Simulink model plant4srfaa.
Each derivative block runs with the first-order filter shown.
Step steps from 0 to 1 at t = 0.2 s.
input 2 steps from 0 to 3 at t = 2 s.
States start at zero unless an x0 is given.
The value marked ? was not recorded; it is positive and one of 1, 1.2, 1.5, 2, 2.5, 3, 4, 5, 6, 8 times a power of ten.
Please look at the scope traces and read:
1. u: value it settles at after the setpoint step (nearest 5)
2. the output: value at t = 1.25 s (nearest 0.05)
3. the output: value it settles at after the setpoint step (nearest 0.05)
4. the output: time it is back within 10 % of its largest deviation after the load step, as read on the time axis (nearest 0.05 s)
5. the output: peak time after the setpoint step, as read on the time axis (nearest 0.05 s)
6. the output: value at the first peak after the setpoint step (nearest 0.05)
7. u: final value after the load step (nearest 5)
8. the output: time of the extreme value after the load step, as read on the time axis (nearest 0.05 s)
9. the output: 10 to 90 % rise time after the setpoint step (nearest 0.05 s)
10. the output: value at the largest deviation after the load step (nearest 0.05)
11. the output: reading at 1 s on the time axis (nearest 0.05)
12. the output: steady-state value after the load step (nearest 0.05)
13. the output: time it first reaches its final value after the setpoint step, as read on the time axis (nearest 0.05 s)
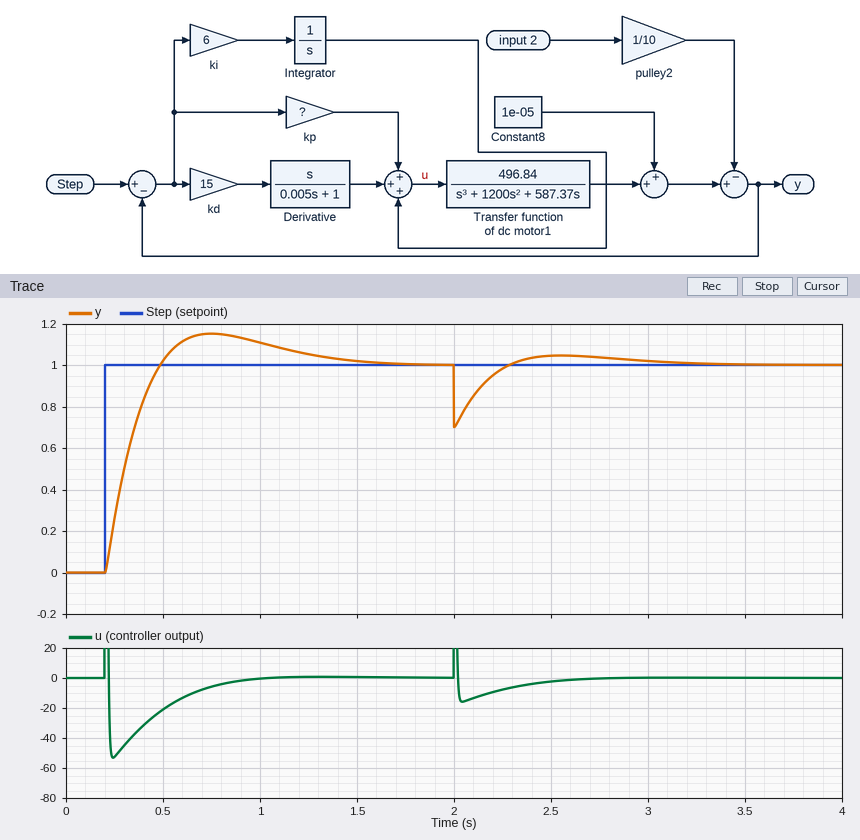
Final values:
0
1.05
1.00
2.85 s
0.75 s
1.15
0
2.00 s
0.20 s
0.70
1.10
1.00
0.50 s
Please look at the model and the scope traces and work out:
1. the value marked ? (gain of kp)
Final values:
40
